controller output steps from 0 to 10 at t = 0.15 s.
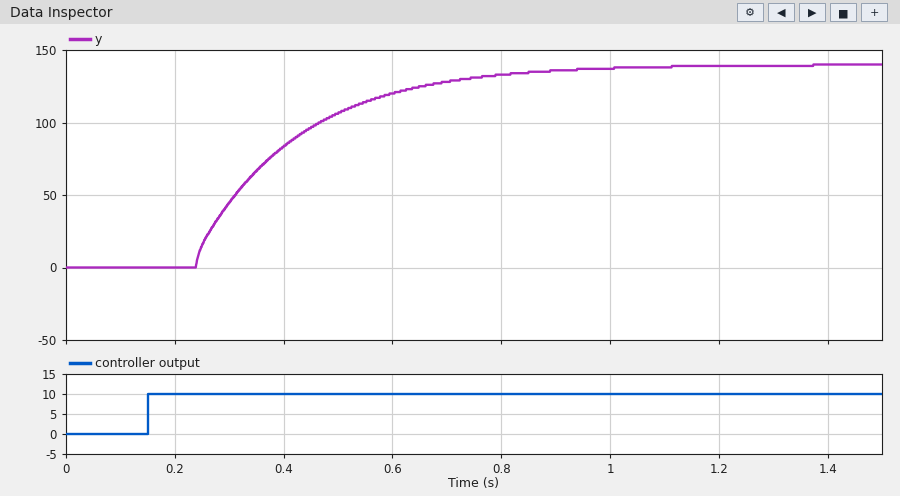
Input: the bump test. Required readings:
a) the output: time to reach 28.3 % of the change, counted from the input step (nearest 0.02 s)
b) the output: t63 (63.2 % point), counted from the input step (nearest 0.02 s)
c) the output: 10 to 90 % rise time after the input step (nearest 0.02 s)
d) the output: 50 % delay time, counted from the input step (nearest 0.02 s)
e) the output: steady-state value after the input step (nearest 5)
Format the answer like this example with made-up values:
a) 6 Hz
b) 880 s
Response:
a) 0.14 s
b) 0.26 s
c) 0.42 s
d) 0.20 s
e) 140
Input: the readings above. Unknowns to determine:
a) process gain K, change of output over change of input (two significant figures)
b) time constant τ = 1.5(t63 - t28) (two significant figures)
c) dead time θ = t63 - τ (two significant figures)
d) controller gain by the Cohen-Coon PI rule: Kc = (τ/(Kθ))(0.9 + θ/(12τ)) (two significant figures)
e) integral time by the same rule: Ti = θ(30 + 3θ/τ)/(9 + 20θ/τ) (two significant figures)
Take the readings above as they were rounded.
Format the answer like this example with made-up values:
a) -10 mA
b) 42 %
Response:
a) 14
b) 0.18 s
c) 0.080 s
d) 0.15
e) 0.14 s
